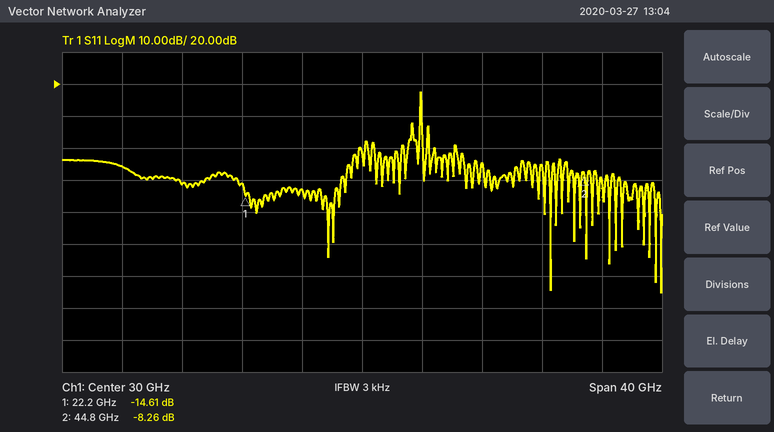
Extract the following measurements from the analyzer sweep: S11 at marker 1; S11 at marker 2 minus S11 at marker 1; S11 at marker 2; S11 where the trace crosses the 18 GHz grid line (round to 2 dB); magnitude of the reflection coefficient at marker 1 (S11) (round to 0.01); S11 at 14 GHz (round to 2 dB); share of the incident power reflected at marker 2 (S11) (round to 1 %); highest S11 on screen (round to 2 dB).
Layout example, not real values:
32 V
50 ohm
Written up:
-14.61 dB
6.35 dB
-8.26 dB
-12 dB
0.19
-6 dB
15 %
18 dB
